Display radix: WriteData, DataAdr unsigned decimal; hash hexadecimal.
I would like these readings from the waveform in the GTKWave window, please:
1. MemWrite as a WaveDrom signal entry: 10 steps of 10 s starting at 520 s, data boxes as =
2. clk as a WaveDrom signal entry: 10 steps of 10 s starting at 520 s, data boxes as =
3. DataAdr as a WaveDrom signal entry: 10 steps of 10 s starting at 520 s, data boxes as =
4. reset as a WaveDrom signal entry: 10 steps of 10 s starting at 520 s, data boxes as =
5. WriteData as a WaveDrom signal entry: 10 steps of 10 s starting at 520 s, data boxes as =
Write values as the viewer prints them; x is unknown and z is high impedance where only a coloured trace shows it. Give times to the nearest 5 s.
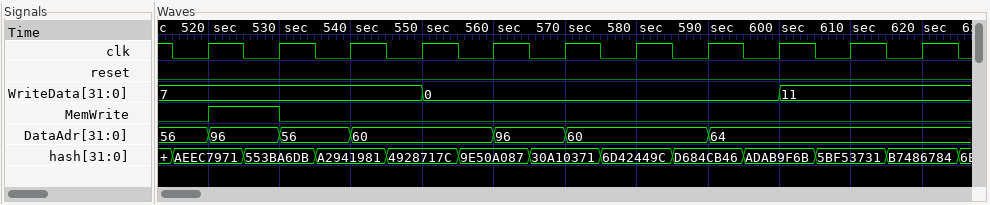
{name: 'MemWrite', wave: '10........'}
{name: 'clk', wave: 'p.........'}
{name: 'DataAdr', wave: '===.==.=..', data: '96 56 60 96 60 64'}
{name: 'reset', wave: '0.........'}
{name: 'WriteData', wave: '=..=....=.', data: '7 0 11'}
